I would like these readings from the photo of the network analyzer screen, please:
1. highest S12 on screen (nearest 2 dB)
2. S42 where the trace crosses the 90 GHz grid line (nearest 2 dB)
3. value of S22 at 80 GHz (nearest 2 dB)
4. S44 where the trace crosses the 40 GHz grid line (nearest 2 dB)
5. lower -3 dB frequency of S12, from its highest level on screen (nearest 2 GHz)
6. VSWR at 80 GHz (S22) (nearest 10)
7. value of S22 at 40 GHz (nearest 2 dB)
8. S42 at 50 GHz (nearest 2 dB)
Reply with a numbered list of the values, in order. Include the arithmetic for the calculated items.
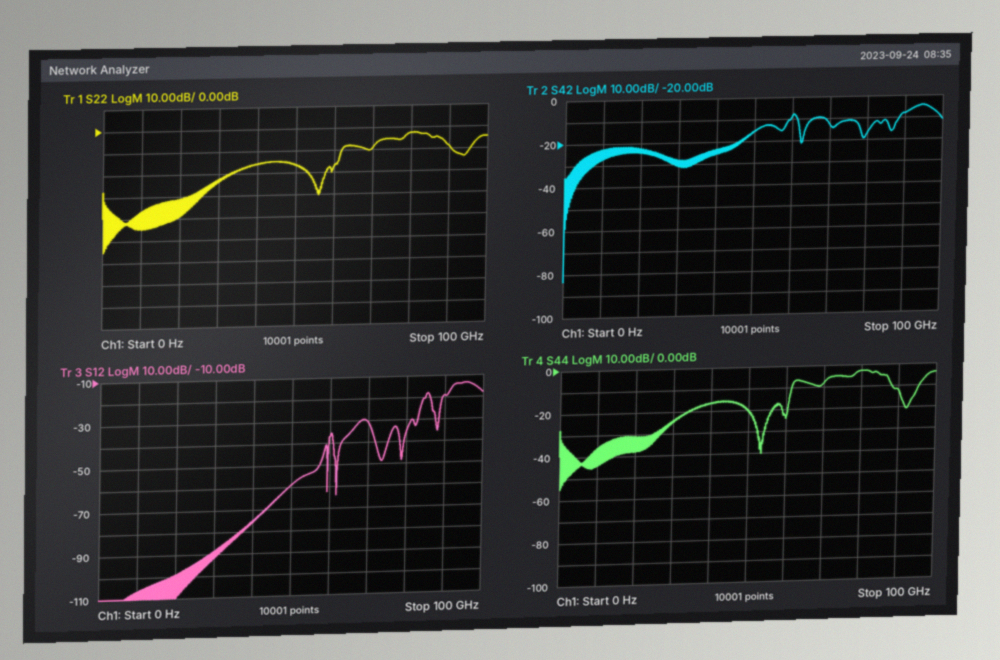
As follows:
1. -14 dB
2. -8 dB
3. -2 dB
4. -16 dB
5. 92 GHz
6. |Γ| = 10^(-2/20) = 0.7943; VSWR = (1 + 0.7943)/(1 − 0.7943) ≈ 8.72, so 10 to the nearest 10
7. -16 dB
8. -16 dB
